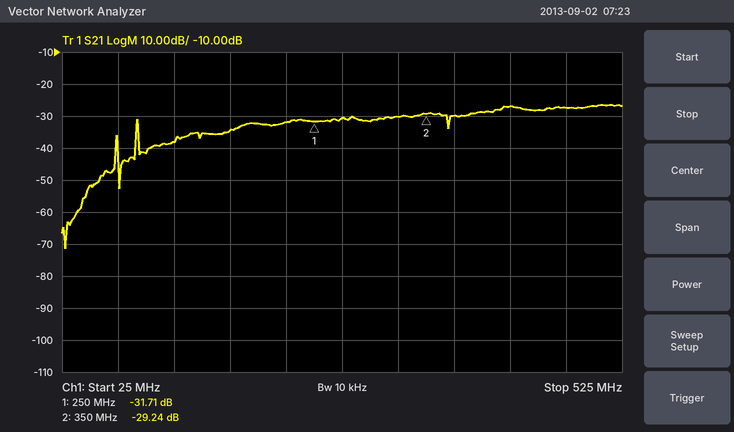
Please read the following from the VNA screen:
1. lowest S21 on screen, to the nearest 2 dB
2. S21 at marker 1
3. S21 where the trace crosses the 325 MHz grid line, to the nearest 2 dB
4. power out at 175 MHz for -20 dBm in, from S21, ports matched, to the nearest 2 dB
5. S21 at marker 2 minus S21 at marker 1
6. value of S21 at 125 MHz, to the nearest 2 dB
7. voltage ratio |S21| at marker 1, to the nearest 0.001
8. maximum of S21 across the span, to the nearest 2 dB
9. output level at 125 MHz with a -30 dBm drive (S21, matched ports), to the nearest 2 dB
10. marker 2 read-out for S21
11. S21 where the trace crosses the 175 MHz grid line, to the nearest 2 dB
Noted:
-72 dB
-31.71 dB
-30 dB
-54 dBm
2.47 dB
-38 dB
0.026
-26 dB
-68 dBm
-29.24 dB
-34 dB
